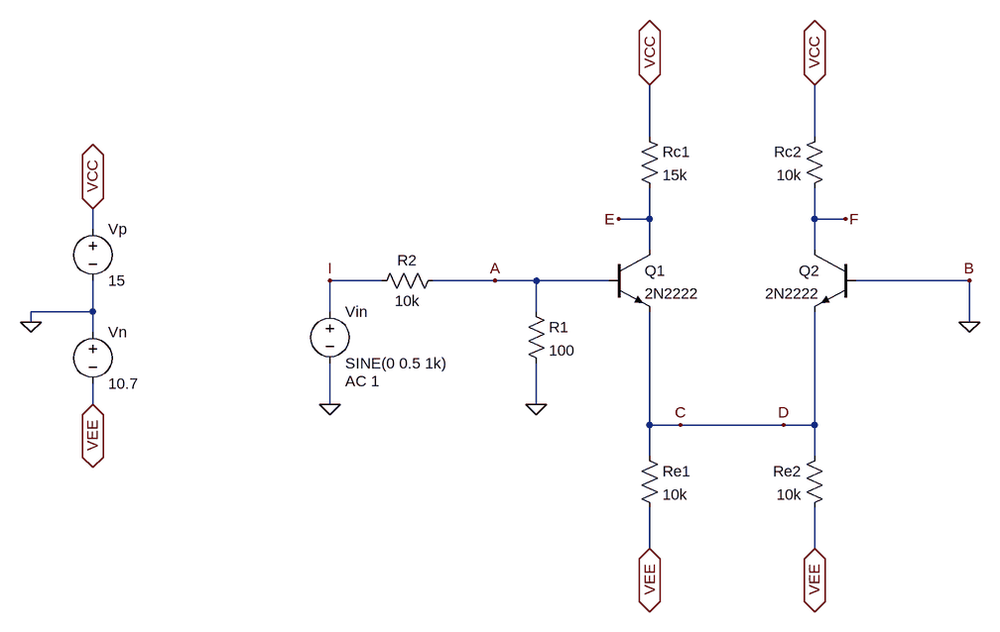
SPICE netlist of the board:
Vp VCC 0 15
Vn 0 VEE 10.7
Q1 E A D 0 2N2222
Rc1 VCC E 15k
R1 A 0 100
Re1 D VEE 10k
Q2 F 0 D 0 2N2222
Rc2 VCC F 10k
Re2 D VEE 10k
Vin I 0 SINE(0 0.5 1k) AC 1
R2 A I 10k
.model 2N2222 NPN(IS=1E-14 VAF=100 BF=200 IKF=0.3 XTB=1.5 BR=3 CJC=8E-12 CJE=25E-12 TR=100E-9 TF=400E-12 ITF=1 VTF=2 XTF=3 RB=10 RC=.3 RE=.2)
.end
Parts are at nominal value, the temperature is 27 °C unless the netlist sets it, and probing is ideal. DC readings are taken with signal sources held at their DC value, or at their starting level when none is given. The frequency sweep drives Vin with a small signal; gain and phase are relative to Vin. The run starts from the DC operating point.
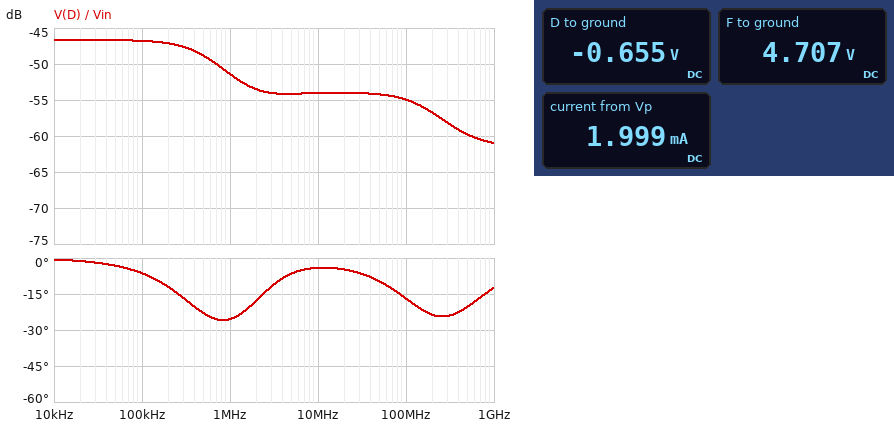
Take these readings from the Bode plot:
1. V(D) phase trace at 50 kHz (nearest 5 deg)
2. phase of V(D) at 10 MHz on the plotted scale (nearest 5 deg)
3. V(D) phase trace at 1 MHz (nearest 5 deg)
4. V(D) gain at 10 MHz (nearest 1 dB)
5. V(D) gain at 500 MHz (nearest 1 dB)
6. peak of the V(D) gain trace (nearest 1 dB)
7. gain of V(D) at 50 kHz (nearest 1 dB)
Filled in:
-5 deg
-5 deg
-25 deg
-54 dB
-60 dB
-47 dB
-47 dB
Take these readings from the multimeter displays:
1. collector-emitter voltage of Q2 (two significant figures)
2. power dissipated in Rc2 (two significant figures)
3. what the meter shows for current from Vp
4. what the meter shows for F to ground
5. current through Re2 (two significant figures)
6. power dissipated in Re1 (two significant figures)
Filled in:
5.4 V
11 mW
1.999 mA
4.707 V
1.0 mA
10 mW
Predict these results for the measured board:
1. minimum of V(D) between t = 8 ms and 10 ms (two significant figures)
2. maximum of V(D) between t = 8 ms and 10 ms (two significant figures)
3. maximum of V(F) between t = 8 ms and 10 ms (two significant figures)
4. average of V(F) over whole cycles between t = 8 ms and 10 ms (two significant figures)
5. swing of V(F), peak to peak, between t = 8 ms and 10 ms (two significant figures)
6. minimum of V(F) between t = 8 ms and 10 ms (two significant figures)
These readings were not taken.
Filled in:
-660 mV
-650 mV
5.4 V
4.7 V
1.5 V
3.9 V
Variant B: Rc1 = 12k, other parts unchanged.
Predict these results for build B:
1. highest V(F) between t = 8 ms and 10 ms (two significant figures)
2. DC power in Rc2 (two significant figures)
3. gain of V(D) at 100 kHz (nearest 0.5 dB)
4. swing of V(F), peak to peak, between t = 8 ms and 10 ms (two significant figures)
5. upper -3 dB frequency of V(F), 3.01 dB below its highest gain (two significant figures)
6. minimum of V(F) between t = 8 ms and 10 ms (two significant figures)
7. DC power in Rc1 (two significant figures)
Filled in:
5.7 V
10 mW
-46.5 dB
1.7 V
1.0 MHz
4.0 V
12 mW
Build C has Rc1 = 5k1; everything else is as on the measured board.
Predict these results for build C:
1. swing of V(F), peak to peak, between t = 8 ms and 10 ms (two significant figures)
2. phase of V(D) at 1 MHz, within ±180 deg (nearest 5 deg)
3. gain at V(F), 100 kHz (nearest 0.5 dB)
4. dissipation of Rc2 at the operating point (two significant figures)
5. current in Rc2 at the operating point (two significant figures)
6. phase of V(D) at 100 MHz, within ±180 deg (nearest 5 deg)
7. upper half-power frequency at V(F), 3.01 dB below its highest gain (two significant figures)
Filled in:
1.7 V
-10 deg
5.0 dB
9.7 mW
990 µA
-20 deg
2.1 MHz
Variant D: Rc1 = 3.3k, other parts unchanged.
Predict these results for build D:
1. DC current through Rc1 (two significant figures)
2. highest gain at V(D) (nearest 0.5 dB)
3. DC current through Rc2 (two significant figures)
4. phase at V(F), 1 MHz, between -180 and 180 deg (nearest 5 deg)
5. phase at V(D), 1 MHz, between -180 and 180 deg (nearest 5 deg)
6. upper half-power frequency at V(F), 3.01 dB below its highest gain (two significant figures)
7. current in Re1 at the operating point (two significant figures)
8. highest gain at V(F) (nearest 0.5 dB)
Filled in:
1.0 mA
-46.0 dB
980 µA
-25 deg
-5 deg
2.6 MHz
1.0 mA
5.0 dB
